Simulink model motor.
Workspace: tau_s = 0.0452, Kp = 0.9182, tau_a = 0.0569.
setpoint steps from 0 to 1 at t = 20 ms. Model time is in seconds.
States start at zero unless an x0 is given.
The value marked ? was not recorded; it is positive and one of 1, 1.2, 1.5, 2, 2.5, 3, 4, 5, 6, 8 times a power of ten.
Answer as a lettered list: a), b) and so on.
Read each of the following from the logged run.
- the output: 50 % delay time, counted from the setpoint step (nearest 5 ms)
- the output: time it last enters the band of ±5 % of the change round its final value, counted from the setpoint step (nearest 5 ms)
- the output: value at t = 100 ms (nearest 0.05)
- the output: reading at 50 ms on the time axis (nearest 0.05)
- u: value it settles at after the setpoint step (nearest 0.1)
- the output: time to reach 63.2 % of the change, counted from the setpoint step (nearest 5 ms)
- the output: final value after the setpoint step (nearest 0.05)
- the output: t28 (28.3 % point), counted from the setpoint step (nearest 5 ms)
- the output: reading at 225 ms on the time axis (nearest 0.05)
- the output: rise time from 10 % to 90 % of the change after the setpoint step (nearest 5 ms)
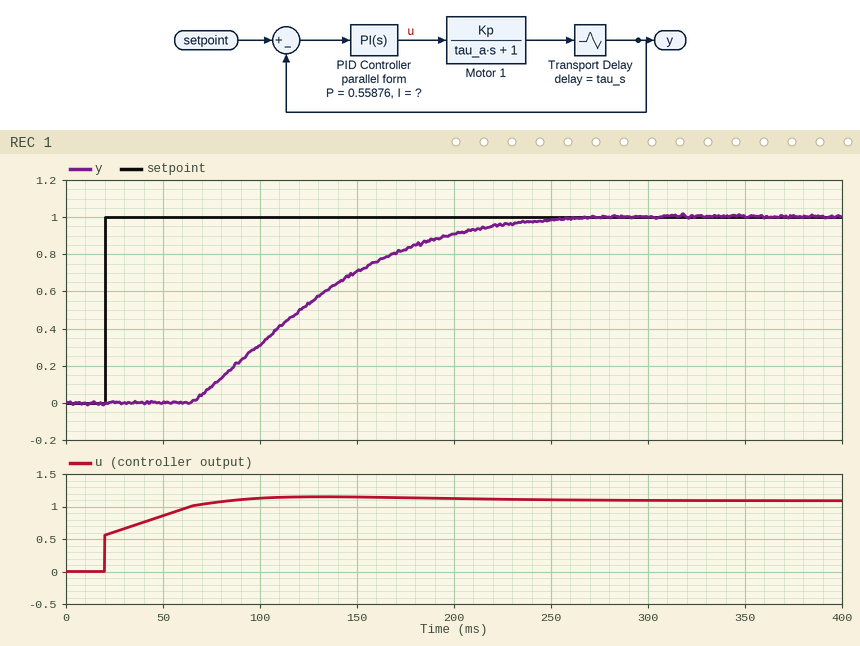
a) 100 ms
b) 200 ms
c) 0.30
d) 0.00
e) 1.1
f) 120 ms
g) 1.00
h) 75 ms
i) 0.95
j) 120 ms
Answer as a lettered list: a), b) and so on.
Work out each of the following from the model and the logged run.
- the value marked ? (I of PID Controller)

a) 10
